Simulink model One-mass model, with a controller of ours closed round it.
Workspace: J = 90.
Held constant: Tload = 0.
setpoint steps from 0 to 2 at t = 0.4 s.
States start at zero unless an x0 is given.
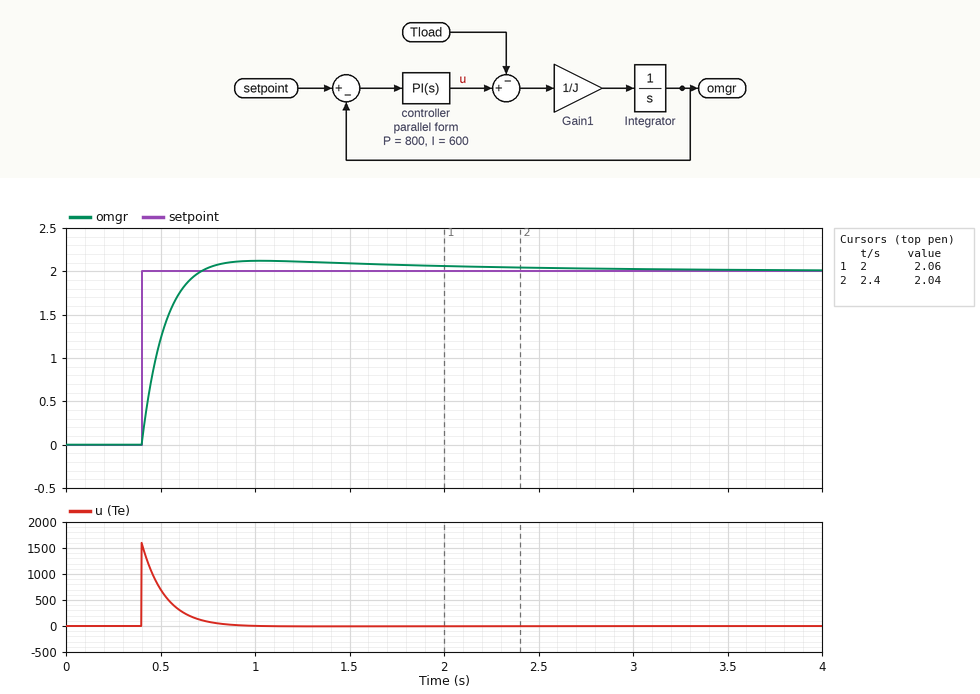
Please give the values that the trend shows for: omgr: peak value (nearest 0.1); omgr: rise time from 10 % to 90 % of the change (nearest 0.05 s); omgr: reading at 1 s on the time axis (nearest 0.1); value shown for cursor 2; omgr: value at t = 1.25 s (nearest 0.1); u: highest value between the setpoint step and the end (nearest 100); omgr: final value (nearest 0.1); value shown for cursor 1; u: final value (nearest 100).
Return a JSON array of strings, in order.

["2.1", "0.20 s", "2.1", "2.04", "2.1", "1600", "2.0", "2.06", "0"]
